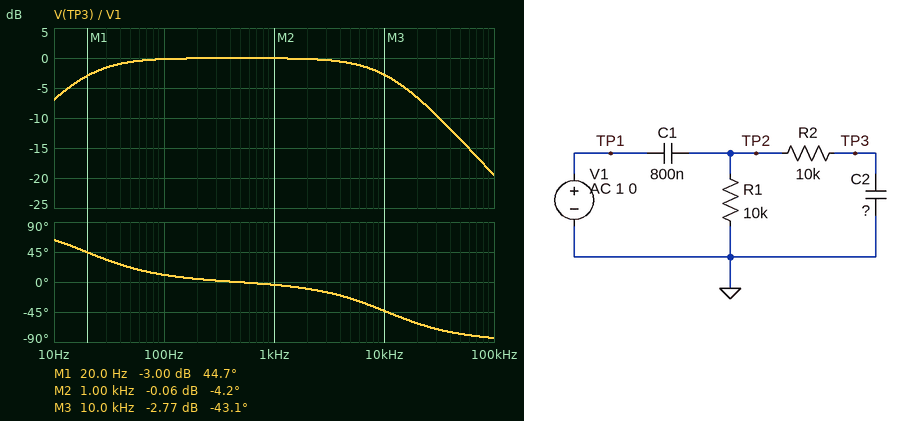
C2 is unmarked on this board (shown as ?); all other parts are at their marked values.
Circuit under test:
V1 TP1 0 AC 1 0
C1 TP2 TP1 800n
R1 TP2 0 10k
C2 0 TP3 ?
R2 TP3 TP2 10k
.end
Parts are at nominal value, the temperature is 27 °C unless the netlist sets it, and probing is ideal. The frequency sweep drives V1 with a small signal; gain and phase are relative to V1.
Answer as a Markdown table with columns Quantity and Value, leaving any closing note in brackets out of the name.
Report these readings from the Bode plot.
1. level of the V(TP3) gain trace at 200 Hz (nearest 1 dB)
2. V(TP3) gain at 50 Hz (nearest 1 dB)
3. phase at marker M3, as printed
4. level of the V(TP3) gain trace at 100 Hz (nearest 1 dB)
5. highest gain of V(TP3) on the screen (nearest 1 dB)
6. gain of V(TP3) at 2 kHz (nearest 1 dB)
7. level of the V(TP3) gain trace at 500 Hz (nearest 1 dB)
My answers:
| Quantity | Value |
|---|---|
| level of the V(TP3) gain trace at 200 Hz | 0 dB |
| V(TP3) gain at 50 Hz | -1 dB |
| phase at marker M3, as printed | -43.1 deg |
| level of the V(TP3) gain trace at 100 Hz | 0 dB |
| highest gain of V(TP3) on the screen | 0 dB |
| gain of V(TP3) at 2 kHz | 0 dB |
| level of the V(TP3) gain trace at 500 Hz | 0 dB |
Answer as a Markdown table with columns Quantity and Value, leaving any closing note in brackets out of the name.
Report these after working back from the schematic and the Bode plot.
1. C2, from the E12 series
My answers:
| Quantity | Value |
|---|---|
| C2, from the E12 series | 1.5 nF |
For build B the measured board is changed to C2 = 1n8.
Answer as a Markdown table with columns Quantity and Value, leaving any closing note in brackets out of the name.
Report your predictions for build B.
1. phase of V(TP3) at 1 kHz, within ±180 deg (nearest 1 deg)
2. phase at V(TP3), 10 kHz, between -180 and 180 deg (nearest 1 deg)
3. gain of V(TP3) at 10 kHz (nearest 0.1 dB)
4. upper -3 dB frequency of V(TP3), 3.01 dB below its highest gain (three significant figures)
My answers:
| Quantity | Value |
|---|---|
| phase of V(TP3) at 1 kHz, within ±180 deg | -5 deg |
| phase at V(TP3), 10 kHz, between -180 and 180 deg | -48 deg |
| gain of V(TP3) at 10 kHz | -3.6 dB |
| upper -3 dB frequency of V(TP3), 3.01 dB below its highest gain | 8.90 kHz |
